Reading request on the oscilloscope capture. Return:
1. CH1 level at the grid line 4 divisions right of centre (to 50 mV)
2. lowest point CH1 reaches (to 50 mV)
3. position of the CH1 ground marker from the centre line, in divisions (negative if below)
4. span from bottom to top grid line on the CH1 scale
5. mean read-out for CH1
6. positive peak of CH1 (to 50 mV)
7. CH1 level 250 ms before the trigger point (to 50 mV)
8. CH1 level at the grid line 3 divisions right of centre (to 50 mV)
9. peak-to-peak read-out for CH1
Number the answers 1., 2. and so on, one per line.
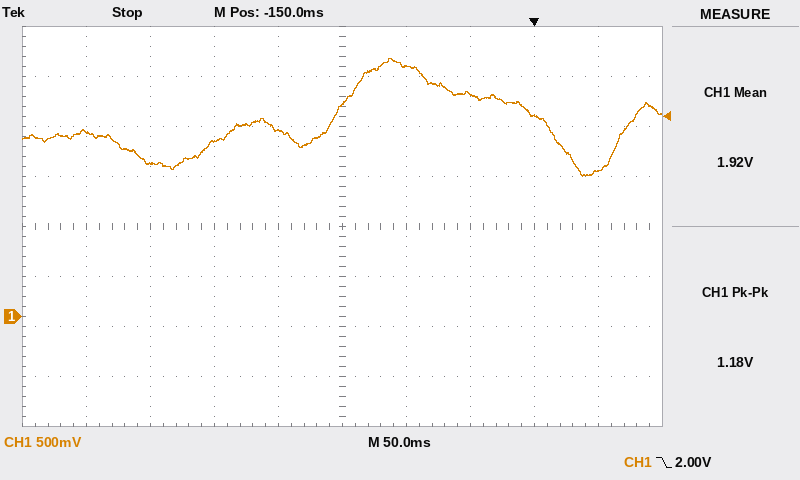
1. 1.45 V
2. 1.40 V
3. -1.8 div
4. 4 V
5. 1.92 V
6. 2.60 V
7. 1.75 V
8. 2.00 V
9. 1.18 V
